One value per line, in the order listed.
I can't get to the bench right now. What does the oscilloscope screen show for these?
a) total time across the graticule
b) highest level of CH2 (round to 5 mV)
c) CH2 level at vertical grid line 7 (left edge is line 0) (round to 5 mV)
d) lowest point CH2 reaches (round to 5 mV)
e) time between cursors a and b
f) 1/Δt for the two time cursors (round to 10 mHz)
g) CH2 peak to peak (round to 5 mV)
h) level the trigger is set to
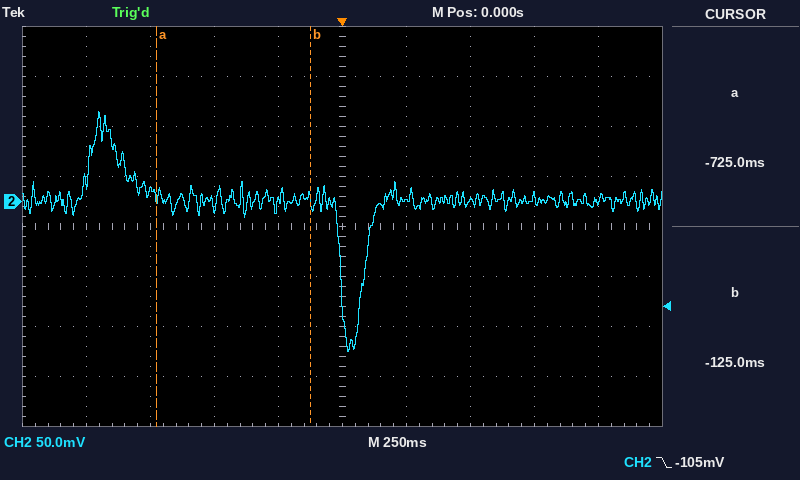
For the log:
2.5 s
90 mV
0 mV
-150 mV
600 ms
1.67 Hz
240 mV
-105 mV
